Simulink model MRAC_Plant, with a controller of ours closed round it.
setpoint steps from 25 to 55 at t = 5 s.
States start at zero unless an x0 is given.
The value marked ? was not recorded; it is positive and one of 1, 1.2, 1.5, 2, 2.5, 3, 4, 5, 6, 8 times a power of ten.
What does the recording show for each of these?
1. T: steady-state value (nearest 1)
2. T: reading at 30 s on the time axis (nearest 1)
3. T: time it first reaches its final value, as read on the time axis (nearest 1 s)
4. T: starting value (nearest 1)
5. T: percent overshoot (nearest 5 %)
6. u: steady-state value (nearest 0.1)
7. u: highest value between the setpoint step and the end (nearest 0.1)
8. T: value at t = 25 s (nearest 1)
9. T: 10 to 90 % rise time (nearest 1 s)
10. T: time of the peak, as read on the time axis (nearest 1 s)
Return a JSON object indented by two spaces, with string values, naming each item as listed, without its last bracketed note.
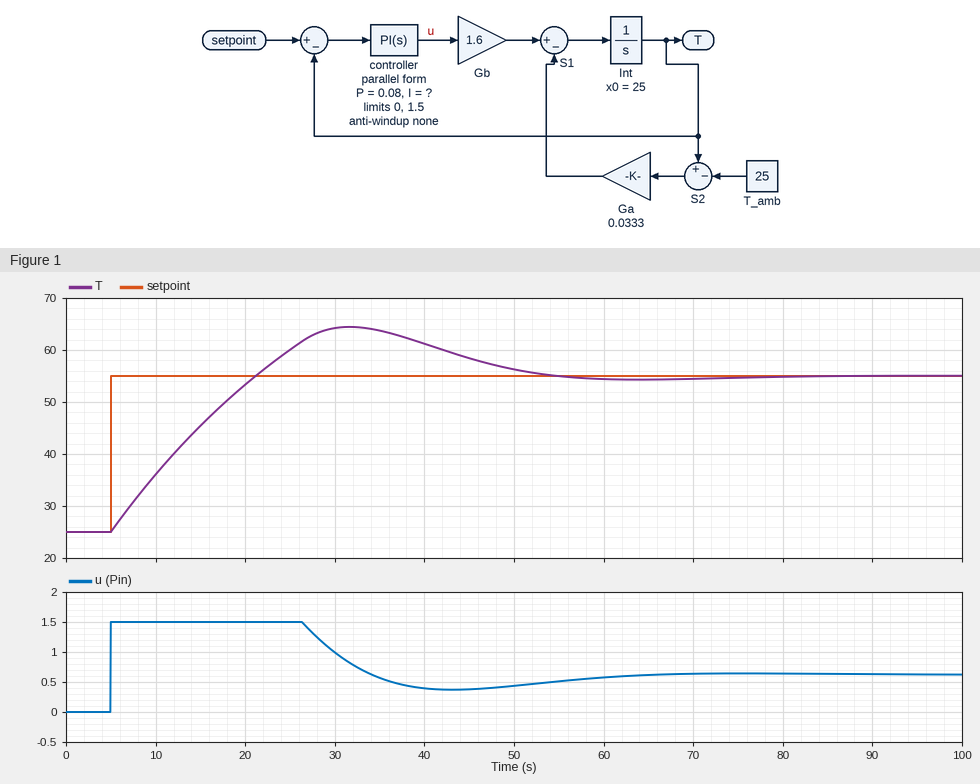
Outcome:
{
  "T: steady-state value": "55",
  "T: reading at 30 s on the time axis": "64",
  "T: time it first reaches its final value, as read on the time axis": "21 s",
  "T: starting value": "25",
  "T: percent overshoot": "30 %",
  "u: steady-state value": "0.6",
  "u: highest value between the setpoint step and the end": "1.5",
  "T: value at t = 25 s": "60",
  "T: 10 to 90 % rise time": "13 s",
  "T: time of the peak, as read on the time axis": "32 s"
}
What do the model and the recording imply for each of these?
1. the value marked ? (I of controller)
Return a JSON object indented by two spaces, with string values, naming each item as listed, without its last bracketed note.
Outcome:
{
  "the value marked ?": "0.01"
}
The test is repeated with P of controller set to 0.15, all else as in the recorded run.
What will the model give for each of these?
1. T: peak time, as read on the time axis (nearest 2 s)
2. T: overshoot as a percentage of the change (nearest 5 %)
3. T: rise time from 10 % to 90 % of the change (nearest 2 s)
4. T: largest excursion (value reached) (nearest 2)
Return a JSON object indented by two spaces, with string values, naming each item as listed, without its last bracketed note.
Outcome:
{
  "T: peak time, as read on the time axis": "30 s",
  "T: overshoot as a percentage of the change": "25 %",
  "T: rise time from 10 % to 90 % of the change": "12 s",
  "T: largest excursion (value reached)": "62"
}
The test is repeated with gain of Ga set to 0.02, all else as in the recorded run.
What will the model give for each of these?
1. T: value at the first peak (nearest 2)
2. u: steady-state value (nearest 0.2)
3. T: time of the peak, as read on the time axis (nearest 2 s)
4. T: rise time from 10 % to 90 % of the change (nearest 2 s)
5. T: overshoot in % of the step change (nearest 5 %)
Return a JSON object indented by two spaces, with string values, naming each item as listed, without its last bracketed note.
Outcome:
{
  "T: value at the first peak": "66",
  "u: steady-state value": "0.4",
  "T: time of the peak, as read on the time axis": "30 s",
  "T: rise time from 10 % to 90 % of the change": "12 s",
  "T: overshoot in % of the step change": "35 %"
}
